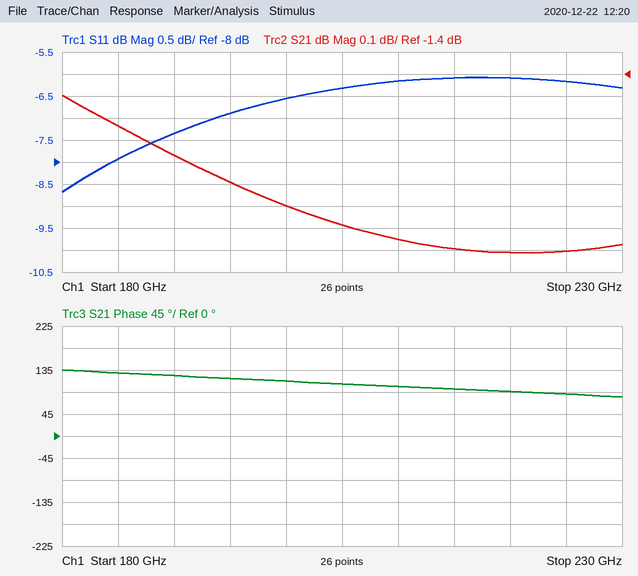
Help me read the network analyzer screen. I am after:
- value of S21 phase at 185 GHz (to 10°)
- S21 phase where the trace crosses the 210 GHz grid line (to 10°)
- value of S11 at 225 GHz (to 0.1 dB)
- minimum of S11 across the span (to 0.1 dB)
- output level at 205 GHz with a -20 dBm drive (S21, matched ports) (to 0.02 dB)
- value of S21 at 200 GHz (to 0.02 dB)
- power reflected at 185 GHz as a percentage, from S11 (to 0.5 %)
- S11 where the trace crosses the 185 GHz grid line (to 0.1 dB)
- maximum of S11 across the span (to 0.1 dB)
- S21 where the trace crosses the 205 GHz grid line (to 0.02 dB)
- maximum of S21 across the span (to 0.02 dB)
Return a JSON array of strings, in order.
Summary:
["130°", "100°", "-6.2 dB", "-8.7 dB", "-22.08 dBm", "-2.00 dB", "16.0 %", "-7.9 dB", "-6.1 dB", "-2.08 dB", "-1.50 dB"]
